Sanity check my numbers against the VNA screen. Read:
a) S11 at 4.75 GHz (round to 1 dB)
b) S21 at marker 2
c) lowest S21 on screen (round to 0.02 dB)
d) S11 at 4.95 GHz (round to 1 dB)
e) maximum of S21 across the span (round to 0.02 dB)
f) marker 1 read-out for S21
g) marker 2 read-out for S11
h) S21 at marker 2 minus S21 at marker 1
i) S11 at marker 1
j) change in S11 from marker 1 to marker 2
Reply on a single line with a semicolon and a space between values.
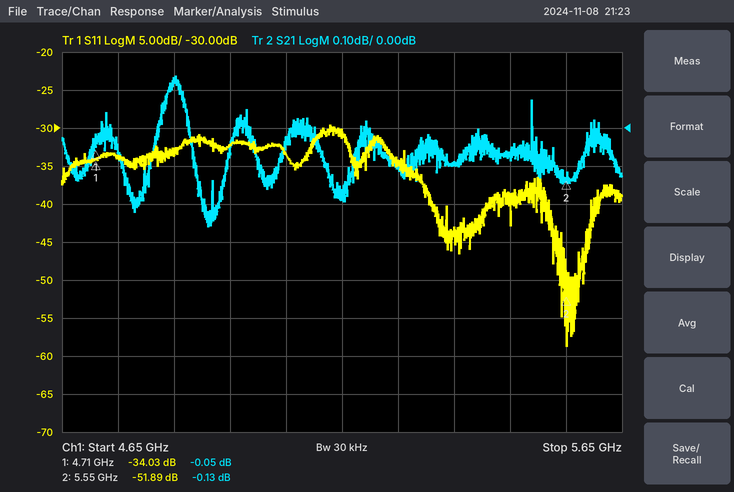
-34 dB; -0.13 dB; -0.26 dB; -32 dB; 0.14 dB; -0.05 dB; -51.89 dB; -0.08 dB; -34.03 dB; -17.86 dB
